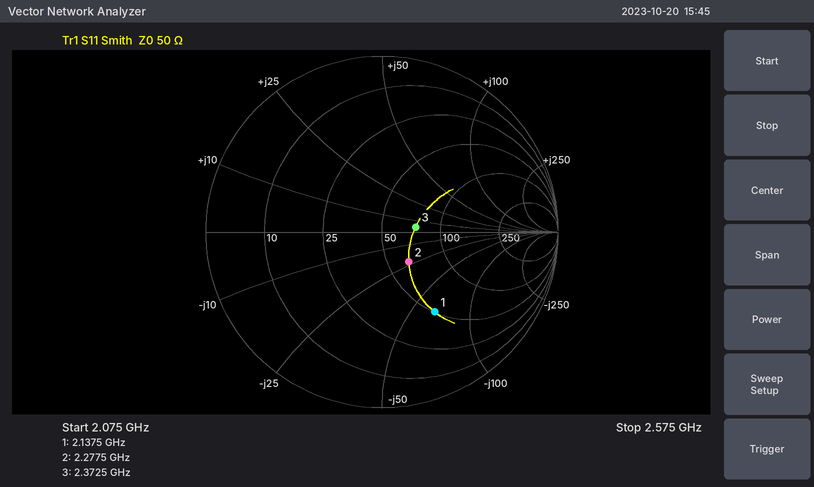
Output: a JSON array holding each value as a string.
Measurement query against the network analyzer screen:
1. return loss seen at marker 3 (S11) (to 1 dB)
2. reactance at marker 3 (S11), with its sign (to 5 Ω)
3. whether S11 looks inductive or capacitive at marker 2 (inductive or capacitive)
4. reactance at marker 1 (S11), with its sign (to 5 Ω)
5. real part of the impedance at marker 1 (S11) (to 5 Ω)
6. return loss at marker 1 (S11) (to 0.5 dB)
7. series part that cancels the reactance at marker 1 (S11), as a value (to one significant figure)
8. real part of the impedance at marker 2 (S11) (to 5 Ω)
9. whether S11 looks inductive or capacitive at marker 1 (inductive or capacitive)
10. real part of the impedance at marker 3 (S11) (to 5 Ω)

["14 dB", "+5 Ω", "capacitive", "-65 Ω", "50 Ω", "5.5 dB", "5 nH", "65 Ω", "capacitive", "75 Ω"]
